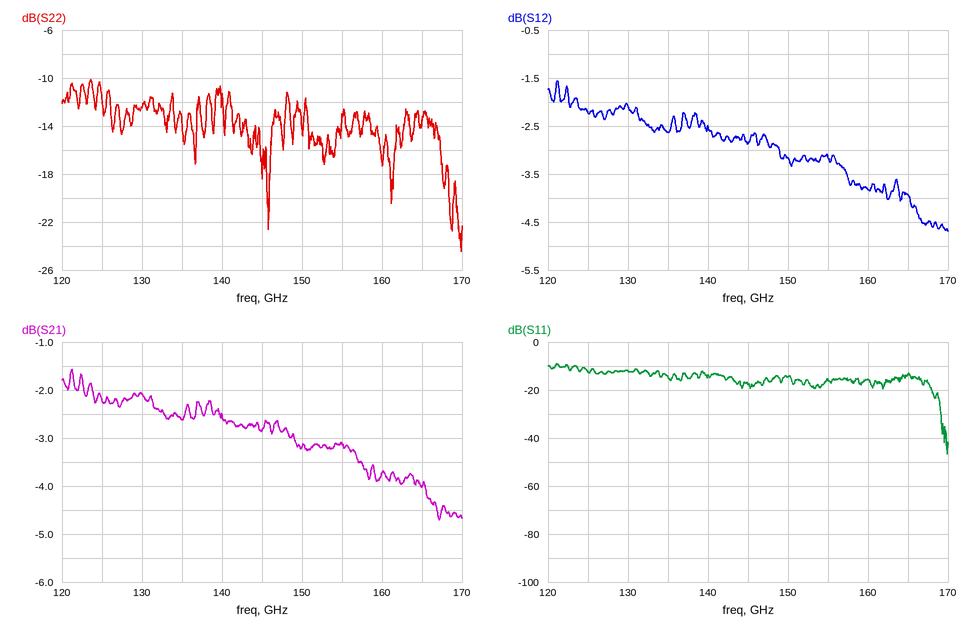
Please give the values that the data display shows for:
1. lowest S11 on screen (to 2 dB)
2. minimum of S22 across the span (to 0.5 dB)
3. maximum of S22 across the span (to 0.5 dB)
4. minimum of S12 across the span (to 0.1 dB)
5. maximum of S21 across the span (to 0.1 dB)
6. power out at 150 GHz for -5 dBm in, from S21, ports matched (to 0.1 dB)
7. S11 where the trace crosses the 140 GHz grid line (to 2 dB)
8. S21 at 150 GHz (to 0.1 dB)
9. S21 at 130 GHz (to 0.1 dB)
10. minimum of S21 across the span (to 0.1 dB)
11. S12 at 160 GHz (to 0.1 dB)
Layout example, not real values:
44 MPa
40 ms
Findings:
-46 dB
-24.5 dB
-10.0 dB
-4.7 dB
-1.6 dB
-8.2 dBm
-14 dB
-3.2 dB
-2.1 dB
-4.7 dB
-3.8 dB
